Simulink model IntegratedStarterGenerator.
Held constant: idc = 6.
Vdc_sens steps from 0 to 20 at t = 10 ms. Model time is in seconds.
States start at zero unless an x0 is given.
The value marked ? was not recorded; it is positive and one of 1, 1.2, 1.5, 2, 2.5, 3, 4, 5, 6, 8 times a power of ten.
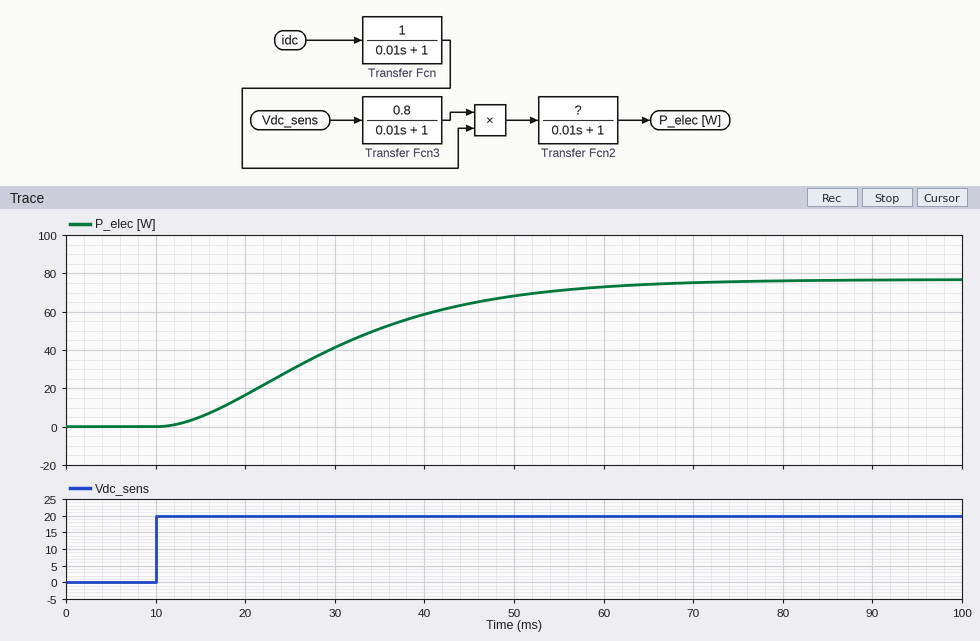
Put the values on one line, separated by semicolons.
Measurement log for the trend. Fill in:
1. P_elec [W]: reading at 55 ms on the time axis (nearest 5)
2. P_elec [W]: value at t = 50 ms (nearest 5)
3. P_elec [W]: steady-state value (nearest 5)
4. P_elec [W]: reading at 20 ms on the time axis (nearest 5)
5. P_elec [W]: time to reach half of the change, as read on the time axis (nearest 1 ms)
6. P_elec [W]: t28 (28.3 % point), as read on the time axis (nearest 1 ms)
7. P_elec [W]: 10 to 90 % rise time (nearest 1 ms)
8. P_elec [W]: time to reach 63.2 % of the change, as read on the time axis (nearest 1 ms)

70; 70; 75; 15; 29 ms; 22 ms; 35 ms; 34 ms
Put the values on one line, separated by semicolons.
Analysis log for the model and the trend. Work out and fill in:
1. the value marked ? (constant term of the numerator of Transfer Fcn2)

0.8
